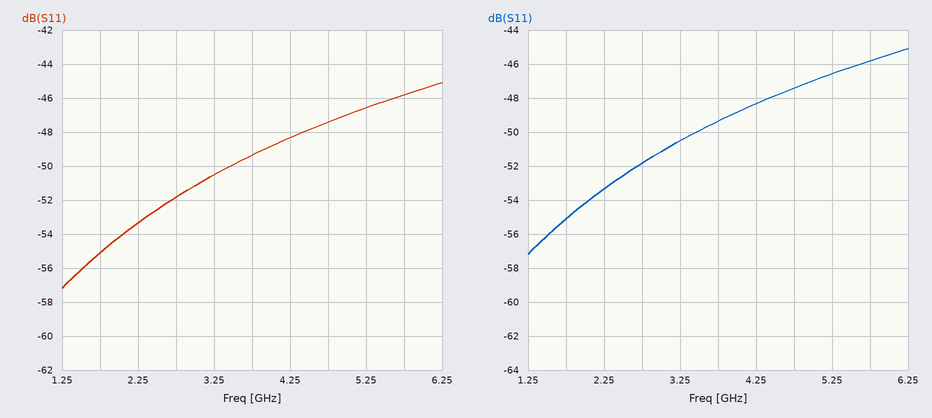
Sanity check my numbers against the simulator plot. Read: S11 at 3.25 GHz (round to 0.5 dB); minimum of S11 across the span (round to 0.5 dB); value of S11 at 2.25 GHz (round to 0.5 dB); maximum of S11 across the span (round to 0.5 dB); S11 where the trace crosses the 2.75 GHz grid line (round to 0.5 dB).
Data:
-50.5 dB
-57.0 dB
-53.5 dB
-45.0 dB
-52.0 dB
